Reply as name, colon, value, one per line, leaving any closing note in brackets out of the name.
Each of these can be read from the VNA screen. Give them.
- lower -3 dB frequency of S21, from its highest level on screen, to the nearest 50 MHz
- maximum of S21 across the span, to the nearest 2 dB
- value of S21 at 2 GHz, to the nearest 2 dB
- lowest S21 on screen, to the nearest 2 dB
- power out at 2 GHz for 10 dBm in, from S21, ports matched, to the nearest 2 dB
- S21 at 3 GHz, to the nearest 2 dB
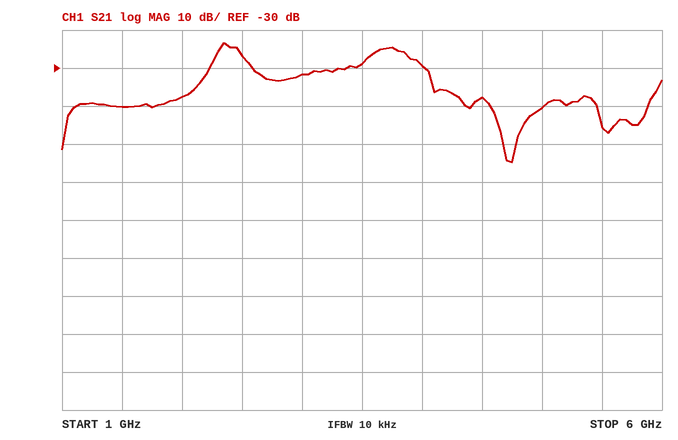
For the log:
lower -3 dB frequency of S21, from its highest level on screen, to the nearest 50 MHz: 2.30 GHz
maximum of S21 across the span, to the nearest 2 dB: -24 dB
value of S21 at 2 GHz, to the nearest 2 dB: -38 dB
lowest S21 on screen, to the nearest 2 dB: -54 dB
power out at 2 GHz for 10 dBm in, from S21, ports matched, to the nearest 2 dB: -28 dBm
S21 at 3 GHz, to the nearest 2 dB: -32 dB
